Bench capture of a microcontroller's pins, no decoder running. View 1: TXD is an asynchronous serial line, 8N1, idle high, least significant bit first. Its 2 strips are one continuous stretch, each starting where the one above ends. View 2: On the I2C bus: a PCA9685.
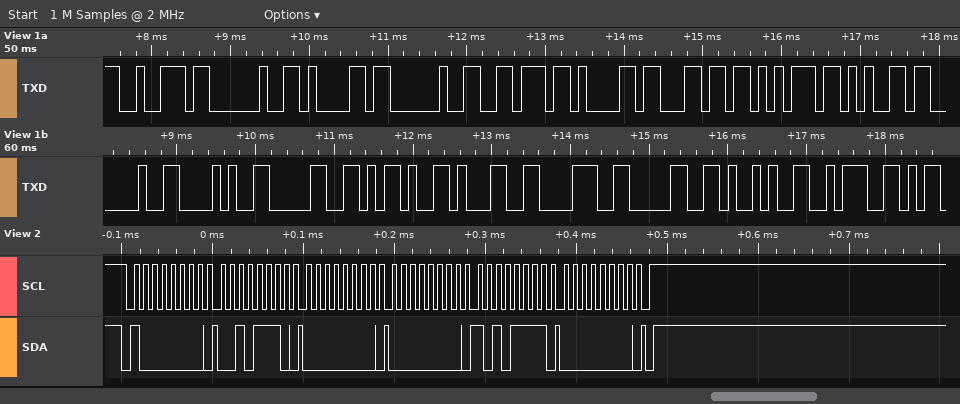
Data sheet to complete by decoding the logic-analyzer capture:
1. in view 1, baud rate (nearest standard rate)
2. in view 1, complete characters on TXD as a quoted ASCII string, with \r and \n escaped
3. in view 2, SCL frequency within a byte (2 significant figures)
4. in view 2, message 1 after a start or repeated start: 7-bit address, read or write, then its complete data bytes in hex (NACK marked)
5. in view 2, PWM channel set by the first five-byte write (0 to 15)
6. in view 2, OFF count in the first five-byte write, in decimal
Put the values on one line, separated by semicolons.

9600 baud; "r a value (0-180):"; 100 kHz; 0x40 write: 2E 00 00 AF 00; 10; 175
